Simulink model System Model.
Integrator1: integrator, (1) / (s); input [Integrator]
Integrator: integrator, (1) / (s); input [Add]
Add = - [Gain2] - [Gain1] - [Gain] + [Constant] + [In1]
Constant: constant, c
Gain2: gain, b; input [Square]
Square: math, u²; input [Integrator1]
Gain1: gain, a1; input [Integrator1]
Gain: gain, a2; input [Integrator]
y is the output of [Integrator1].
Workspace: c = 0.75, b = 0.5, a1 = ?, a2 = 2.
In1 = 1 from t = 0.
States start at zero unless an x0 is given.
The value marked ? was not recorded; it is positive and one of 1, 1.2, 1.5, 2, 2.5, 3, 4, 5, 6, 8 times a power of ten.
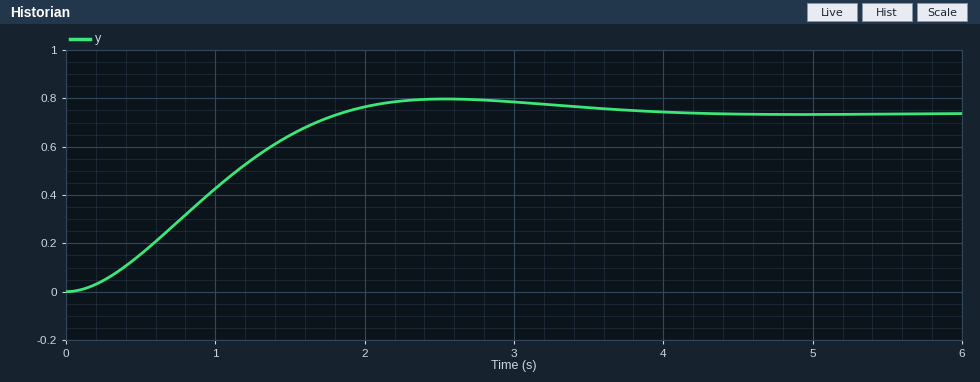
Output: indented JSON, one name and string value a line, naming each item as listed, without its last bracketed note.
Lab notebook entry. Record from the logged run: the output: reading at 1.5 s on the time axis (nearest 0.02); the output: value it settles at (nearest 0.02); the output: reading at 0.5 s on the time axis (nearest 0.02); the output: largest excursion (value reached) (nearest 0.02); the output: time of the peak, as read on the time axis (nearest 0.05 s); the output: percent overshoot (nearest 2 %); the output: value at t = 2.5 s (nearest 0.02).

{
  "the output: reading at 1.5 s on the time axis": "0.64",
  "the output: value it settles at": "0.74",
  "the output: reading at 0.5 s on the time axis": "0.16",
  "the output: largest excursion (value reached)": "0.80",
  "the output: time of the peak, as read on the time axis": "2.55 s",
  "the output: percent overshoot": "8 %",
  "the output: value at t = 2.5 s": "0.80"
}
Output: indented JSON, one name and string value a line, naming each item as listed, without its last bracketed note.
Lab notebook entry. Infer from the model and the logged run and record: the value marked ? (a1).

{
  "the value marked ?": "2"
}
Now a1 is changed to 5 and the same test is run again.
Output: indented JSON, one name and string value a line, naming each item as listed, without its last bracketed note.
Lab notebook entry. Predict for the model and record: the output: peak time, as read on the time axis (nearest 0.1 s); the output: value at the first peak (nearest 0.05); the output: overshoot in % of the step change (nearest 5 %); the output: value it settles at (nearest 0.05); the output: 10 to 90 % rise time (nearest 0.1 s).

{
  "the output: peak time, as read on the time axis": "1.5 s",
  "the output: value at the first peak": "0.40",
  "the output: overshoot in % of the step change": "20 %",
  "the output: value it settles at": "0.35",
  "the output: 10 to 90 % rise time": "0.7 s"
}
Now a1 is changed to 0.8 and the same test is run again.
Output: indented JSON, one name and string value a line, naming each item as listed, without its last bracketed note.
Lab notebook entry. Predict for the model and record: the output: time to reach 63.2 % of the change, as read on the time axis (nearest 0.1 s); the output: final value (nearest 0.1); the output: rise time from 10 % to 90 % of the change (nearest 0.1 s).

{
  "the output: time to reach 63.2 % of the change, as read on the time axis": "1.5 s",
  "the output: final value": "1.2",
  "the output: rise time from 10 % to 90 % of the change": "1.9 s"
}
